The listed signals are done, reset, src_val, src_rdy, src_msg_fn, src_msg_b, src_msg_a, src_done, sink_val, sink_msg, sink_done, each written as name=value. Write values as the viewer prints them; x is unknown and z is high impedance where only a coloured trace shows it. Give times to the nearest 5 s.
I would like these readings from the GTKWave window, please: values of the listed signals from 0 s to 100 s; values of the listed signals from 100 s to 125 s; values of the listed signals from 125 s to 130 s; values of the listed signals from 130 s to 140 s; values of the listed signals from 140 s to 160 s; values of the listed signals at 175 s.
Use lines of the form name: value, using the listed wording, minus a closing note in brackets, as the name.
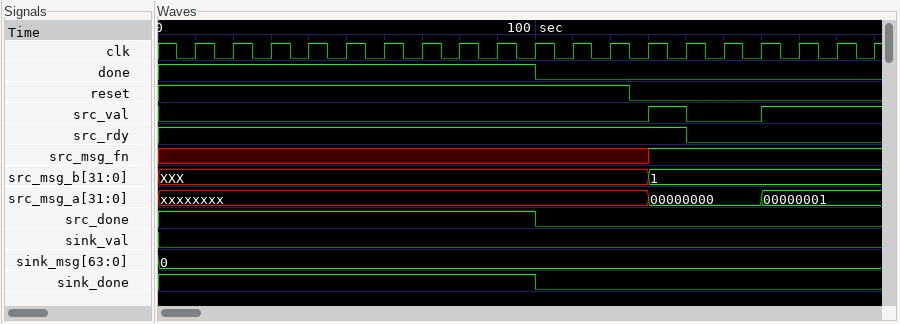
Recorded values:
values of the listed signals from 0 s to 100 s: done=1, reset=1, src_val=0, src_rdy=1, src_msg_fn=x, src_msg_b=XXX, src_msg_a=xxxxxxxx, src_done=1, sink_val=0, sink_msg=0, sink_done=1
values of the listed signals from 100 s to 125 s: done=0, reset=1, src_val=0, src_rdy=1, src_msg_fn=x, src_msg_b=XXX, src_msg_a=xxxxxxxx, src_done=0, sink_val=0, sink_msg=0, sink_done=0
values of the listed signals from 125 s to 130 s: done=0, reset=0, src_val=0, src_rdy=1, src_msg_fn=x, src_msg_b=XXX, src_msg_a=xxxxxxxx, src_done=0, sink_val=0, sink_msg=0, sink_done=0
values of the listed signals from 130 s to 140 s: done=0, reset=0, src_val=1, src_rdy=1, src_msg_fn=1, src_msg_b=1, src_msg_a=00000000, src_done=0, sink_val=0, sink_msg=0, sink_done=0
values of the listed signals from 140 s to 160 s: done=0, reset=0, src_val=0, src_rdy=0, src_msg_fn=1, src_msg_b=1, src_msg_a=00000000, src_done=0, sink_val=0, sink_msg=0, sink_done=0
values of the listed signals at 175 s: done=0, reset=0, src_val=1, src_rdy=0, src_msg_fn=1, src_msg_b=1, src_msg_a=00000001, src_done=0, sink_val=0, sink_msg=0, sink_done=0
